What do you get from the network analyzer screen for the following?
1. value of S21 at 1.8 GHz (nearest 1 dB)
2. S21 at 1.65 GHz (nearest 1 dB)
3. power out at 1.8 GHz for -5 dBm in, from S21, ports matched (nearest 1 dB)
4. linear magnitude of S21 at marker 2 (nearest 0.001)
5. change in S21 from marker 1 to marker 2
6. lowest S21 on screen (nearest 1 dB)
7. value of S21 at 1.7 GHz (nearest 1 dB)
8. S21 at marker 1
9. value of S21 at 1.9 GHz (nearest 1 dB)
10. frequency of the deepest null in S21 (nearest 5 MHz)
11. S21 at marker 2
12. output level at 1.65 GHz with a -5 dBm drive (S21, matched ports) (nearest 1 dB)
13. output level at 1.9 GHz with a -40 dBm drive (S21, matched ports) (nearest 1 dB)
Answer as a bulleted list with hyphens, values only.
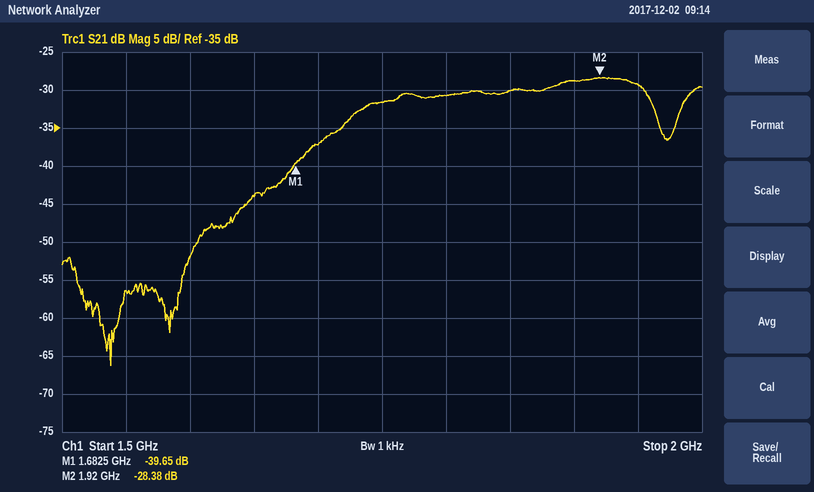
- -31 dB
- -44 dB
- -36 dBm
- 0.038
- 11.27 dB
- -66 dB
- -37 dB
- -39.65 dB
- -29 dB
- 1.540 GHz
- -28.38 dB
- -49 dBm
- -69 dBm
